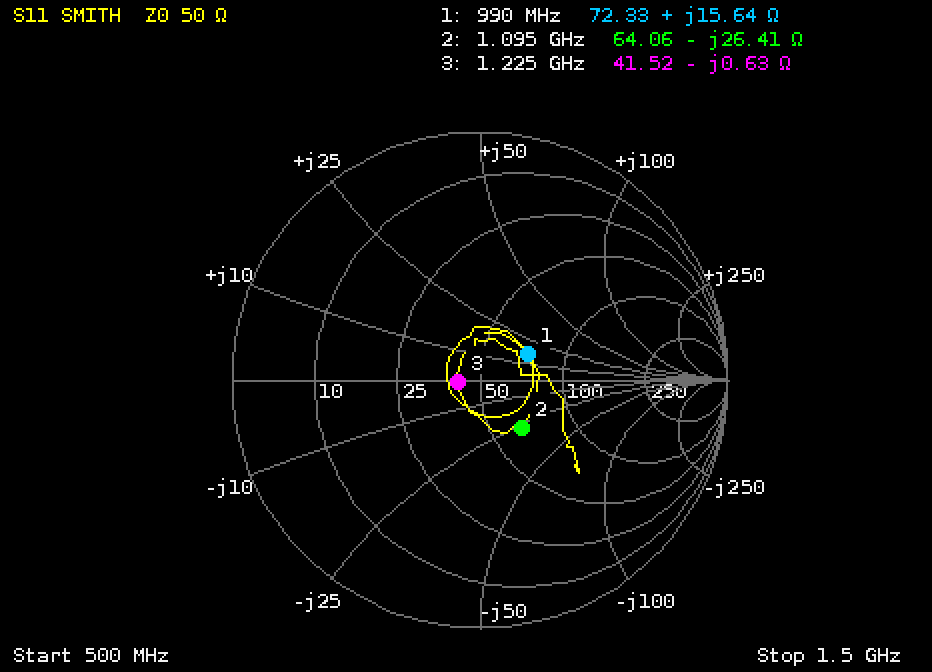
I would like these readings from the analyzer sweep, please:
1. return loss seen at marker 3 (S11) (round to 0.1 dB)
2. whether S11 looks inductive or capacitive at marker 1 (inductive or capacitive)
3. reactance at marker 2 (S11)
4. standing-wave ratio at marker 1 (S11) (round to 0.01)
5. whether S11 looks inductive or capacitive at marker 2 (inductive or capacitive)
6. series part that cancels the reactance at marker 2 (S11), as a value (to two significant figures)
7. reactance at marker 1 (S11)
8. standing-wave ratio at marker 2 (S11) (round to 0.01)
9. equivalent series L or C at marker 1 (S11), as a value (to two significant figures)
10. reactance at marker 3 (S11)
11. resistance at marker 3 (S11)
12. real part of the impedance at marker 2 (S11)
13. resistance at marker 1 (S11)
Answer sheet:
20.6 dB
inductive
-26.41 Ω
1.57
capacitive
3.8 nH
+15.64 Ω
1.69
2.5 nH
-0.63 Ω
41.52 Ω
64.06 Ω
72.33 Ω
